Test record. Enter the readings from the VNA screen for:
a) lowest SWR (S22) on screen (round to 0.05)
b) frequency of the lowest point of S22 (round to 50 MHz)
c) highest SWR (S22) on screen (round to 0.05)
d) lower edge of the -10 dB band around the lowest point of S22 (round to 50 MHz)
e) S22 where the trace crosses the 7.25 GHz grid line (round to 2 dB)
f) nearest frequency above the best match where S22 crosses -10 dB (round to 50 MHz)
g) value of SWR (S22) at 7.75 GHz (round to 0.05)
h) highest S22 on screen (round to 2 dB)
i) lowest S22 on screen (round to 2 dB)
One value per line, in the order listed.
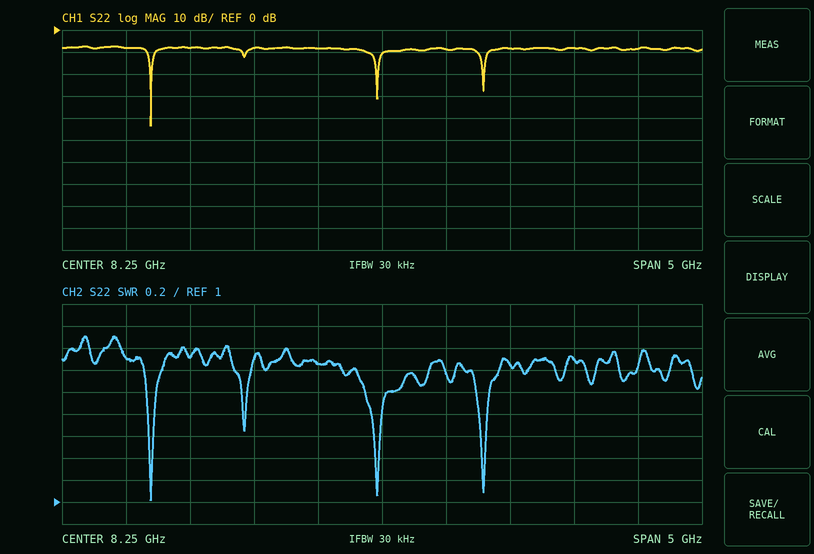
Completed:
1.00
6.45 GHz
2.50
6.40 GHz
-8 dB
6.50 GHz
2.25
-8 dB
-44 dB
